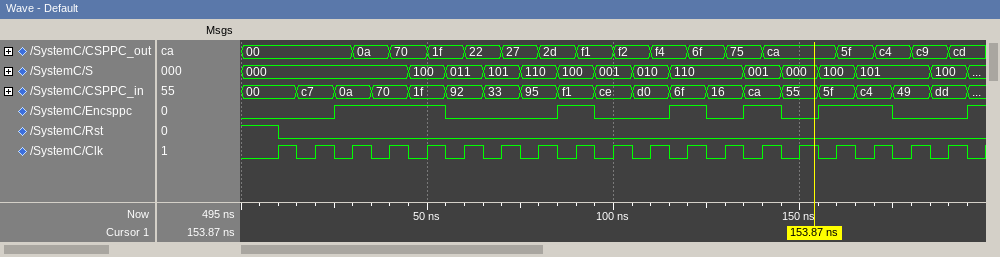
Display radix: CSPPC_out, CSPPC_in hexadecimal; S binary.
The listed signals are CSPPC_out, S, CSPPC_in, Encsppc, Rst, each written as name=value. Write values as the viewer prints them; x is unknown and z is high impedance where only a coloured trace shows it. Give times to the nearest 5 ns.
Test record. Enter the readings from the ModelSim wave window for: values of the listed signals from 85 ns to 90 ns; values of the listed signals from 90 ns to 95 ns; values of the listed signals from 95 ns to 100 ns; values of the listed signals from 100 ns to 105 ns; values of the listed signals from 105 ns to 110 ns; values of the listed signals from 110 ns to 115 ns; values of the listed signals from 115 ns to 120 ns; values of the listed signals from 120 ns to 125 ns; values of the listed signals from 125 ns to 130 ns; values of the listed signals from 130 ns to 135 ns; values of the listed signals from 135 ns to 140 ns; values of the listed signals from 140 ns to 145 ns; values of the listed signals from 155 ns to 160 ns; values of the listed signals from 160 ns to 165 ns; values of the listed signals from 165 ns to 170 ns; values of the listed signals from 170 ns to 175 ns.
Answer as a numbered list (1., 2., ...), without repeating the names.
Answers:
1. CSPPC_out=2d, S=100, CSPPC_in=f1, Encsppc=1, Rst=0
2. CSPPC_out=f1, S=100, CSPPC_in=f1, Encsppc=1, Rst=0
3. CSPPC_out=f1, S=001, CSPPC_in=ce, Encsppc=0, Rst=0
4. CSPPC_out=f2, S=001, CSPPC_in=ce, Encsppc=0, Rst=0
5. CSPPC_out=f2, S=010, CSPPC_in=d0, Encsppc=0, Rst=0
6. CSPPC_out=f4, S=010, CSPPC_in=d0, Encsppc=0, Rst=0
7. CSPPC_out=f4, S=110, CSPPC_in=6f, Encsppc=1, Rst=0
8. CSPPC_out=6f, S=110, CSPPC_in=6f, Encsppc=1, Rst=0
9. CSPPC_out=6f, S=110, CSPPC_in=16, Encsppc=0, Rst=0
10. CSPPC_out=75, S=110, CSPPC_in=16, Encsppc=0, Rst=0
11. CSPPC_out=75, S=001, CSPPC_in=ca, Encsppc=1, Rst=0
12. CSPPC_out=ca, S=001, CSPPC_in=ca, Encsppc=1, Rst=0
13. CSPPC_out=ca, S=100, CSPPC_in=5f, Encsppc=1, Rst=0
14. CSPPC_out=5f, S=100, CSPPC_in=5f, Encsppc=1, Rst=0
15. CSPPC_out=5f, S=101, CSPPC_in=c4, Encsppc=1, Rst=0
16. CSPPC_out=c4, S=101, CSPPC_in=c4, Encsppc=1, Rst=0
